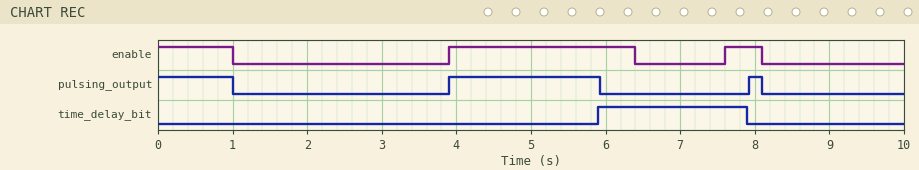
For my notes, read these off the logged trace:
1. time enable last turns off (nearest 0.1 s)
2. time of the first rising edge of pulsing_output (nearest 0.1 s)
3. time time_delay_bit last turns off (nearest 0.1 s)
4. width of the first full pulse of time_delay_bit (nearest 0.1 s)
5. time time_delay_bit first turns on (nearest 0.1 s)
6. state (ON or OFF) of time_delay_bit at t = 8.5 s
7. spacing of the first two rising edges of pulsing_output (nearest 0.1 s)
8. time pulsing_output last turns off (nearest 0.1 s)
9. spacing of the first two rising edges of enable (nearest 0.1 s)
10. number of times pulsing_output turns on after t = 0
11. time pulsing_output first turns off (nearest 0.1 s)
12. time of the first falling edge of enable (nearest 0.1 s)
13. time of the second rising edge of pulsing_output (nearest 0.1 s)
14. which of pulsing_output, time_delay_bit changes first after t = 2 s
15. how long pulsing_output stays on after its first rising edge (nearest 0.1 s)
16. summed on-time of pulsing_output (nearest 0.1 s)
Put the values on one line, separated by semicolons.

8.1 s; 3.9 s; 7.9 s; 2.0 s; 5.9 s; OFF; 4.0 s; 8.1 s; 3.7 s; 2; 1.0 s; 1.0 s; 7.9 s; pulsing_output; 2.0 s; 3.2 s
